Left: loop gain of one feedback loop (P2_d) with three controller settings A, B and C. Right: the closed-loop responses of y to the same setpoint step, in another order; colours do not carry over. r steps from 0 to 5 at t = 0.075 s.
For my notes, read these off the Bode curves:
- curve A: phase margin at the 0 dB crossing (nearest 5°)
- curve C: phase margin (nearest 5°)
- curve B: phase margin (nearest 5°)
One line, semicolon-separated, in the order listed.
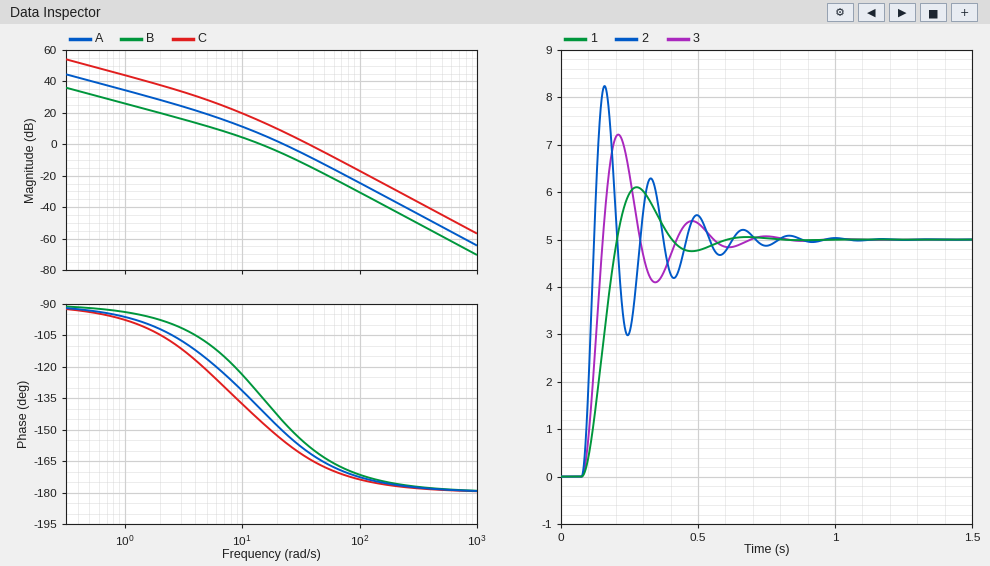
30°; 15°; 45°
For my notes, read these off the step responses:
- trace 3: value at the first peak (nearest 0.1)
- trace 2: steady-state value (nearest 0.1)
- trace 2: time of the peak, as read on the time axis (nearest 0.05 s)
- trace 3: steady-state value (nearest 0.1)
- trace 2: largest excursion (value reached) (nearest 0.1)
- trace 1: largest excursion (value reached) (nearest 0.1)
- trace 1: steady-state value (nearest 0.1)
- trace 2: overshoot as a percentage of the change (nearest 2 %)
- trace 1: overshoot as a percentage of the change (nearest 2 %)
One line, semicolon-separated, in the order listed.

7.2; 5.0; 0.15 s; 5.0; 8.2; 6.1; 5.0; 64 %; 22 %
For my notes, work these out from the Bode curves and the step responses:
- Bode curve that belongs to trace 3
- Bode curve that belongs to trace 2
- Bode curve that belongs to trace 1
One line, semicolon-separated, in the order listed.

A; C; B
